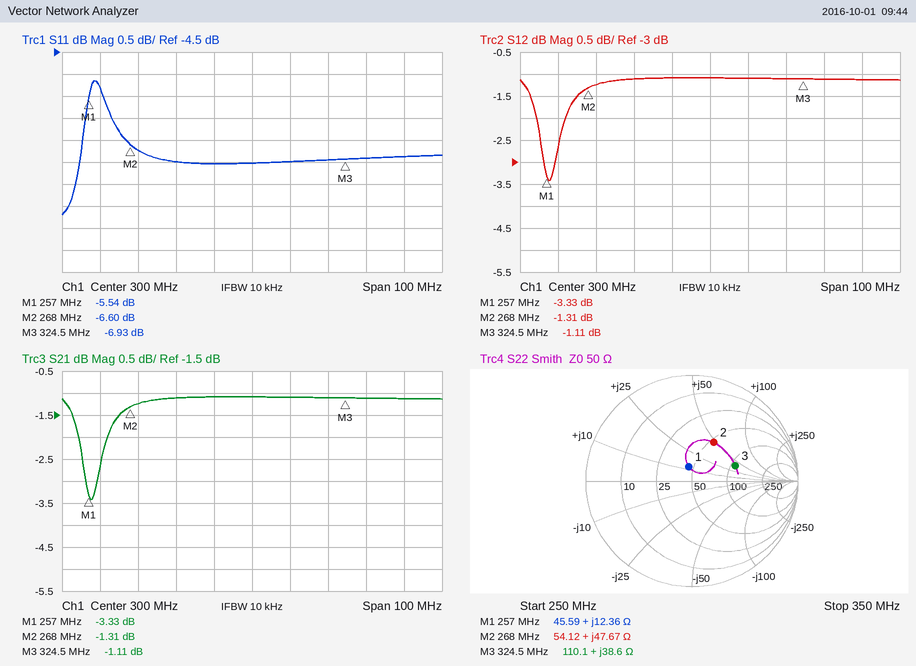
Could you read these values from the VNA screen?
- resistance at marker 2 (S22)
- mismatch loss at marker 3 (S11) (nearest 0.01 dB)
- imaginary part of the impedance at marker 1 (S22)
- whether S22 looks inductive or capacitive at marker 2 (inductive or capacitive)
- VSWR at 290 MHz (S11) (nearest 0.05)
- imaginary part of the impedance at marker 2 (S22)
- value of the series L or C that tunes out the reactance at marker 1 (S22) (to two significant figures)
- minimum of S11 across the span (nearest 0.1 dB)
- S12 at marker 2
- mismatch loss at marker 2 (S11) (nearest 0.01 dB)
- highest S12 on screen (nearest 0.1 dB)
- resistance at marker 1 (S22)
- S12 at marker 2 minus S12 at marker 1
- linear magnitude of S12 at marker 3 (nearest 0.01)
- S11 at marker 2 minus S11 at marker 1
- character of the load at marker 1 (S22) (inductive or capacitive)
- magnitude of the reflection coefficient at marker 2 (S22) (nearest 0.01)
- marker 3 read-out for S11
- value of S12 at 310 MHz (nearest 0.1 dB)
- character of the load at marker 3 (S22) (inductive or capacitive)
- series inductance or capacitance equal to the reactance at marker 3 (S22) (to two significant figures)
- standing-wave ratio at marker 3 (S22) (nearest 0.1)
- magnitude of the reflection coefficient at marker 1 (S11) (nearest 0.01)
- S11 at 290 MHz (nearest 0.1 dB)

54.12 Ω
0.98 dB
+12.36 Ω
inductive
2.60
+47.67 Ω
50 pF
-8.2 dB
-1.31 dB
1.07 dB
-1.1 dB
45.59 Ω
2.02 dB
0.88
-1.06 dB
inductive
0.42
-6.93 dB
-1.1 dB
inductive
19 nH
2.5
0.53
-7.0 dB
